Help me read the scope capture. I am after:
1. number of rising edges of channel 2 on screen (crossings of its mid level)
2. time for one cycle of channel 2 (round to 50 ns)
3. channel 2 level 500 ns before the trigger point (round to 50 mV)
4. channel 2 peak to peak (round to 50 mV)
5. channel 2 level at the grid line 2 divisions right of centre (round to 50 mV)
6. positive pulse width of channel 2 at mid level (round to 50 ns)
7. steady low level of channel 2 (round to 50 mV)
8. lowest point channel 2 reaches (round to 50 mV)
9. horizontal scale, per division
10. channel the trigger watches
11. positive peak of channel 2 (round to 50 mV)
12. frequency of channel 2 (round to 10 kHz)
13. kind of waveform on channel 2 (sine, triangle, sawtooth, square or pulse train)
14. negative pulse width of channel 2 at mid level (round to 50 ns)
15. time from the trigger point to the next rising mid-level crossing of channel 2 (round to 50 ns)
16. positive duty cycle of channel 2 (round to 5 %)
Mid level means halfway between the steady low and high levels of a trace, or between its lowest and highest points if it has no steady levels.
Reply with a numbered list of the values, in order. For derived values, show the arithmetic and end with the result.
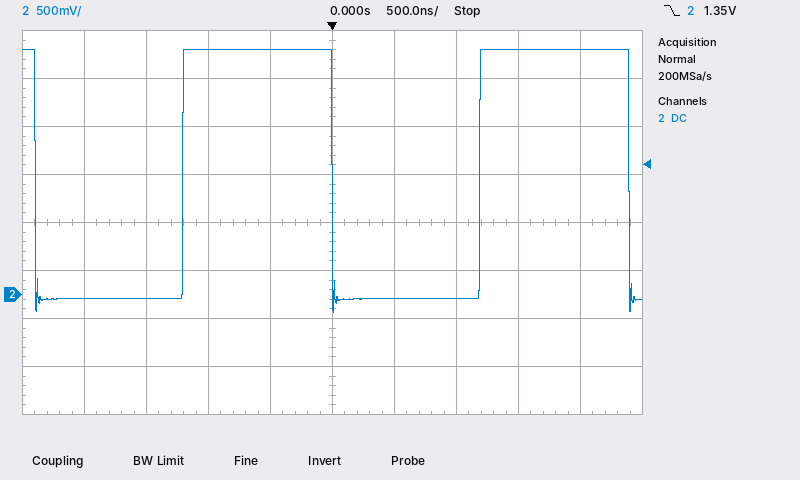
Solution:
1. 2
2. 2.40 µs
3. 2.55 V
4. 2.55 V − (-200 mV) = 2.75 V
5. -50 mV
6. 1.20 µs
7. -50 mV
8. -200 mV
9. 500 ns
10. channel 2
11. 2.55 V
12. 1 / 2.40 µs ≈ 417 kHz, so 420 kHz to the nearest 10 kHz
13. square
14. 1.20 µs
15. 1.20 µs
16. 1.20 µs / 2.40 µs ≈ 50 %
